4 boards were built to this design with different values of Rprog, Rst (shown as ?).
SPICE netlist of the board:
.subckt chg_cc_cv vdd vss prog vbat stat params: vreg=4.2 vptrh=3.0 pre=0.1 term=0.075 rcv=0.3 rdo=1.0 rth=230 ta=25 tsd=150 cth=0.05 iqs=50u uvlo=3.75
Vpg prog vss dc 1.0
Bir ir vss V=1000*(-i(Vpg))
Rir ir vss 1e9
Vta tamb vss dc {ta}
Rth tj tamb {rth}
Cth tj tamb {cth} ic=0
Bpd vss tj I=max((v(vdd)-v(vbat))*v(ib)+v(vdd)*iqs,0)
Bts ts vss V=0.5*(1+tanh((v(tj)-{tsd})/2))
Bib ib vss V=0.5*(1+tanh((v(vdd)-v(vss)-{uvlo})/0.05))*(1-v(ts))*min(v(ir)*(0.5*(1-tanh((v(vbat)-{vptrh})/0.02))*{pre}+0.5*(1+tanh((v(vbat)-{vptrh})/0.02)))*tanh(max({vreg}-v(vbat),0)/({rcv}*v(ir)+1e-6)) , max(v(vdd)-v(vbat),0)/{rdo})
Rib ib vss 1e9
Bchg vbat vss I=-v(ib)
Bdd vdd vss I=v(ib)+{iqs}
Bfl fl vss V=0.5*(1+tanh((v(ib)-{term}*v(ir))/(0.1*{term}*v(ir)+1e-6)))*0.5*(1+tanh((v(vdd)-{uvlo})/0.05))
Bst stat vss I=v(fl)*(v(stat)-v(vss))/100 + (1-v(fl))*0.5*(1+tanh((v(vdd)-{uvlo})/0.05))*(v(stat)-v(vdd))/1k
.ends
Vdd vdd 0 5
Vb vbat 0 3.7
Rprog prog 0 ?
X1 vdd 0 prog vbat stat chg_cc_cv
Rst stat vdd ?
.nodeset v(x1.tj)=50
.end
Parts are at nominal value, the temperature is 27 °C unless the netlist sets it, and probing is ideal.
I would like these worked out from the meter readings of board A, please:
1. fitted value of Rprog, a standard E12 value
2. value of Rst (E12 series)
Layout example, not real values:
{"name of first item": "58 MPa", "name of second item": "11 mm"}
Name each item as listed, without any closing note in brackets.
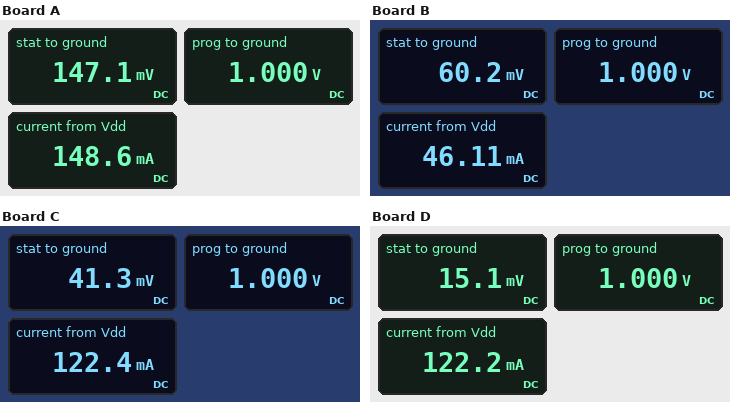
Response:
{"fitted value of Rprog, a standard E12 value": "6.8 kΩ", "value of Rst": "3.3 kΩ"}
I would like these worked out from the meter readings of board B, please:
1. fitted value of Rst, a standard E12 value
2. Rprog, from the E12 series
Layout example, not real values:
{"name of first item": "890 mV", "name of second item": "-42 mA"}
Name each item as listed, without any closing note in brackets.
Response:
{"fitted value of Rst, a standard E12 value": "8.2 kΩ", "Rprog, from the E12 series": "22 kΩ"}
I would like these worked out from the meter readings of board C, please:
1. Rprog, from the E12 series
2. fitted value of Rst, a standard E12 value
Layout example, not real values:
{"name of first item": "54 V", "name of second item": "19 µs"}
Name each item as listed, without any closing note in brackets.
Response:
{"Rprog, from the E12 series": "8.2 kΩ", "fitted value of Rst, a standard E12 value": "12 kΩ"}
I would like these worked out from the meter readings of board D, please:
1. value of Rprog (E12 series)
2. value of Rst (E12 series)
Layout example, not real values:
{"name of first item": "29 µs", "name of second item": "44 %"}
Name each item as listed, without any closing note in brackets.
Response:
{"value of Rprog": "8.2 kΩ", "value of Rst": "33 kΩ"}
